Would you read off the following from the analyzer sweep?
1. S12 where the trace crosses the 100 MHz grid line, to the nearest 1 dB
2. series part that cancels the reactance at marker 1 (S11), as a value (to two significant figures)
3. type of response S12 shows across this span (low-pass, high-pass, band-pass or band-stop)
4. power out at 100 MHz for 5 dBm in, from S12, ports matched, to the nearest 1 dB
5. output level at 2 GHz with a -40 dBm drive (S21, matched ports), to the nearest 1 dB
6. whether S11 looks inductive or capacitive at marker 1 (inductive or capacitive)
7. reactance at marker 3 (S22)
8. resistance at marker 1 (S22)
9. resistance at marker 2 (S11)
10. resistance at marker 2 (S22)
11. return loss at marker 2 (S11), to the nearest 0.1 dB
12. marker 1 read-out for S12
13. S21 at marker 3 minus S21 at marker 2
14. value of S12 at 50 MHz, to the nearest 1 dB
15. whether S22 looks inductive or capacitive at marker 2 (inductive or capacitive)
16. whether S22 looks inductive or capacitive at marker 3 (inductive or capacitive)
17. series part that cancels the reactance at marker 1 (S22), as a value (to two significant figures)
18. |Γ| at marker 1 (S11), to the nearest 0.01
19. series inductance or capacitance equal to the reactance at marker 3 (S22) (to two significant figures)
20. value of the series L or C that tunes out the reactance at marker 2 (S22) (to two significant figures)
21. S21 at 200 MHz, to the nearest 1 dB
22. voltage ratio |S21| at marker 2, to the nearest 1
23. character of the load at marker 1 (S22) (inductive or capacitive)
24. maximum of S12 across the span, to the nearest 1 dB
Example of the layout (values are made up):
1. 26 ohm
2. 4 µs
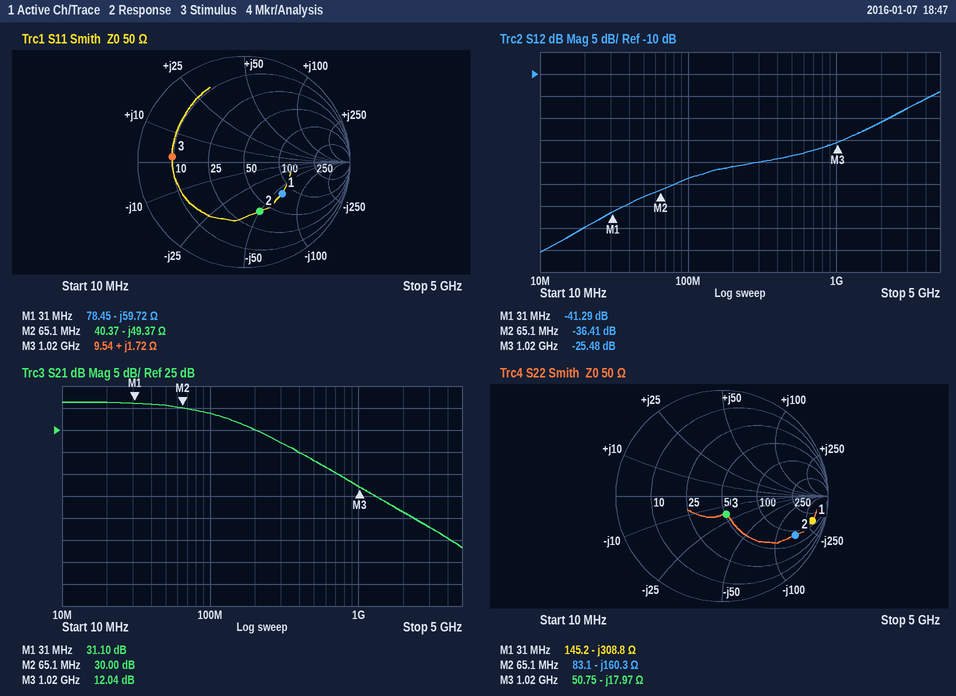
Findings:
1. -34 dB
2. 310 nH
3. high-pass
4. -29 dBm
5. -34 dBm
6. capacitive
7. -17.97 Ω
8. 145.2 Ω
9. 40.37 Ω
10. 83.1 Ω
11. 6.2 dB
12. -41.29 dB
13. -17.96 dB
14. -38 dB
15. capacitive
16. capacitive
17. 1.6 µH
18. 0.47
19. 8.7 pF
20. 390 nH
21. 25 dB
22. 32
23. capacitive
24. -14 dB
